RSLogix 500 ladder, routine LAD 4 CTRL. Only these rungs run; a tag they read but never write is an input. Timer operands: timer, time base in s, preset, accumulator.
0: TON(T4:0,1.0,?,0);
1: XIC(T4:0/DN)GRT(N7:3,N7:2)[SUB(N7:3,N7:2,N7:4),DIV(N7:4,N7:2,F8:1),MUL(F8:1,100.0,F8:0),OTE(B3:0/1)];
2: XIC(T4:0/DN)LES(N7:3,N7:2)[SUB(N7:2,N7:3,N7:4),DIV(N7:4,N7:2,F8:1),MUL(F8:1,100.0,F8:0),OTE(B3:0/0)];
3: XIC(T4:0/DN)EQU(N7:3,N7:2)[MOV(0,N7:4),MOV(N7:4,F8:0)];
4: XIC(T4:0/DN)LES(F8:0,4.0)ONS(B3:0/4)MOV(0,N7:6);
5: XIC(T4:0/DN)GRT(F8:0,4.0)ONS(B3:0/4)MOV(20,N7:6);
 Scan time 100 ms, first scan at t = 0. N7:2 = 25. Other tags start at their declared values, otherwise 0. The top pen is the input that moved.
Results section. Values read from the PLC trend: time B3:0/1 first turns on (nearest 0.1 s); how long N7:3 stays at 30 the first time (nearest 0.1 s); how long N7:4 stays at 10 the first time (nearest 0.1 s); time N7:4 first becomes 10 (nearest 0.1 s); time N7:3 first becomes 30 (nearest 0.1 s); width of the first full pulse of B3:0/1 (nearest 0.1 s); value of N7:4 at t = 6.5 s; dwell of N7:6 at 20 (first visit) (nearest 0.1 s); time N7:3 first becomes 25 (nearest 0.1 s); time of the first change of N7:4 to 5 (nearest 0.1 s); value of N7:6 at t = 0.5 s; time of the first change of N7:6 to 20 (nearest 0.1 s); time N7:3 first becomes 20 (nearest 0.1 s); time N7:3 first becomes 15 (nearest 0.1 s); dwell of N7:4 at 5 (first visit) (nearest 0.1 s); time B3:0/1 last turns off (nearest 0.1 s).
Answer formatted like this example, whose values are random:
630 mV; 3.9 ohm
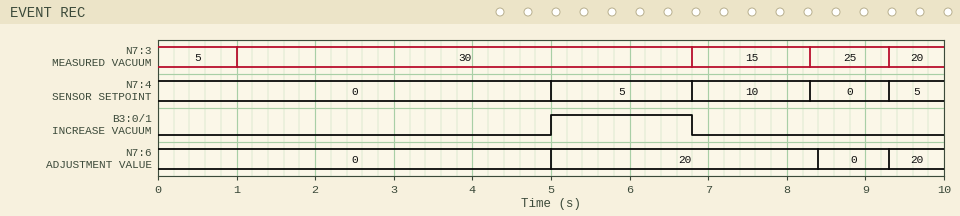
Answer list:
5.0 s; 5.8 s; 1.5 s; 6.8 s; 1.0 s; 1.8 s; 5; 3.4 s; 8.3 s; 5.0 s; 0; 5.0 s; 9.3 s; 6.8 s; 1.8 s; 6.8 s
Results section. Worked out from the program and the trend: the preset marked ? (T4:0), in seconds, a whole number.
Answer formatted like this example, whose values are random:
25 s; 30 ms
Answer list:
5 s
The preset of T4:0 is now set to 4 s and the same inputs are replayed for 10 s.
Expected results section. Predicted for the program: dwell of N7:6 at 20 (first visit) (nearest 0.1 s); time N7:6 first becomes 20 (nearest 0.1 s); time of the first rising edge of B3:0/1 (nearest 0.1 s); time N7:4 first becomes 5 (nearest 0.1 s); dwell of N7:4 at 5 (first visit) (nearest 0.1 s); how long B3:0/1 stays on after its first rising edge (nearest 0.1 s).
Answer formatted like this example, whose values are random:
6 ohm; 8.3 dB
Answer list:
4.4 s; 4.0 s; 4.0 s; 4.0 s; 2.8 s; 2.8 s
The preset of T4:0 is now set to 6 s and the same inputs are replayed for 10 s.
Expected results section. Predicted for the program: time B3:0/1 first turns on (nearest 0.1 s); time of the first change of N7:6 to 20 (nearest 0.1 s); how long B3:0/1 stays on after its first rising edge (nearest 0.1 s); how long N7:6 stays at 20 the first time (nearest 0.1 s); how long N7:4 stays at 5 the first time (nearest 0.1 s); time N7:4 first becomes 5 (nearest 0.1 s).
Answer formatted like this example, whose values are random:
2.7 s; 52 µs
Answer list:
6.0 s; 6.0 s; 0.8 s; 2.4 s; 0.8 s; 6.0 s
